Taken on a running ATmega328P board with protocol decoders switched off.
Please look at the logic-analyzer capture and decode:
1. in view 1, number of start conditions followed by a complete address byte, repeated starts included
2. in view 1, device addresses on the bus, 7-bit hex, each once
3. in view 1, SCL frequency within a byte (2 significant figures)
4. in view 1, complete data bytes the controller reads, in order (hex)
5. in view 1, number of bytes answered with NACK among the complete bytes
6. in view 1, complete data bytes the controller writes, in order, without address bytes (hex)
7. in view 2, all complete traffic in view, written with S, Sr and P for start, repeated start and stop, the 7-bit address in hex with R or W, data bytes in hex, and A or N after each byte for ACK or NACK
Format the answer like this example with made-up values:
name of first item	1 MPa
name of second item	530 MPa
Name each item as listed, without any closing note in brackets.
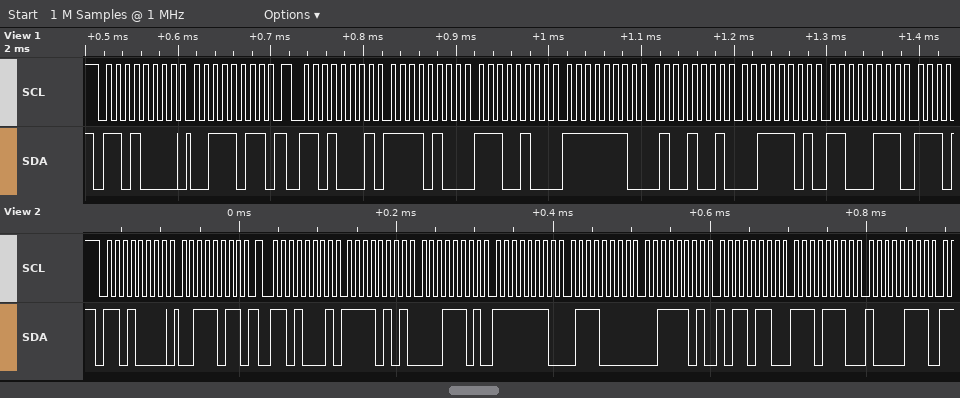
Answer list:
in view 1, number of start conditions followed by a complete address byte, repeated starts included	2
in view 1, device addresses on the bus, 7-bit hex, each once	0x68
in view 1, SCL frequency within a byte	100 kHz
in view 1, complete data bytes the controller reads, in order	F4 E4 FE 49 3D C7
in view 1, number of bytes answered with NACK among the complete bytes	0
in view 1, complete data bytes the controller writes, in order, without address bytes	3B
in view 2, all complete traffic in view, written with S, Sr and P for start, repeated start and stop, the 7-bit address in hex with R or W, data bytes in hex, and A or N after each byte for ACK or NACK	S 68W A 3B A Sr 68R A F5 A 1D A FE A 70 A 3D A B6 A EE A 87 A
